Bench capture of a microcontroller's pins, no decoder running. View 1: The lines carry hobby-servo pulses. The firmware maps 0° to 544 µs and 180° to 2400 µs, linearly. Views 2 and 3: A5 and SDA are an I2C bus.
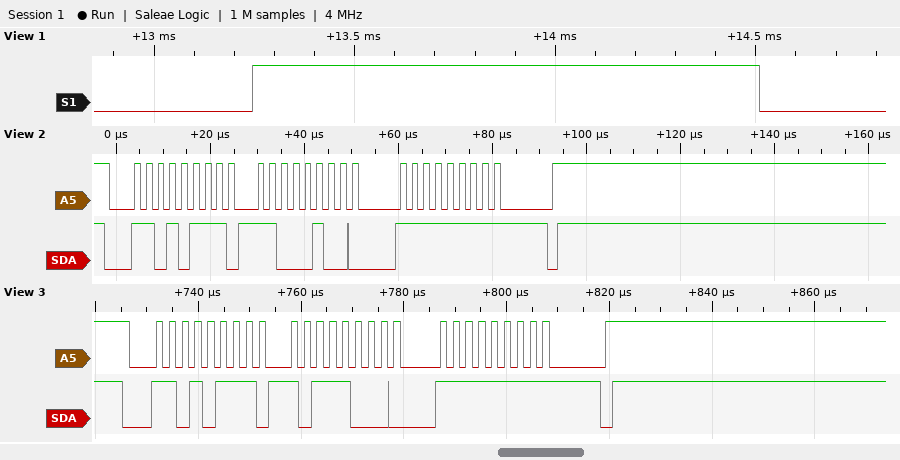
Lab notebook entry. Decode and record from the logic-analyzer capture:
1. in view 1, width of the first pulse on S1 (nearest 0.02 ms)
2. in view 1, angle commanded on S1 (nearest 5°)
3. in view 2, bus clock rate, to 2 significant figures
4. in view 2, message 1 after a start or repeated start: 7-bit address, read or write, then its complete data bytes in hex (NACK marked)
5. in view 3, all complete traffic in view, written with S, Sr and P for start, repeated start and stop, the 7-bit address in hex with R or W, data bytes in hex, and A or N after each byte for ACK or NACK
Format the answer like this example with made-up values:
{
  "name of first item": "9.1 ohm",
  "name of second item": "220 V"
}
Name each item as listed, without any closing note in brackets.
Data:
{
  "in view 1, width of the first pulse on S1": "1.26 ms",
  "in view 1, angle commanded on S1": "70°",
  "in view 2, bus clock rate, to 2 significant figures": "400 kHz",
  "in view 2, message 1 after a start or repeated start: 7-bit address, read or write, then its complete data bytes in hex": "0x6B read: C4 FF NACK",
  "in view 3, all complete traffic in view, written with S, Sr and P for start, repeated start and stop, the 7-bit address in hex with R or W, data bytes in hex, and A or N after each byte for ACK or NACK": "S 6BR A B8 A FF N P"
}
